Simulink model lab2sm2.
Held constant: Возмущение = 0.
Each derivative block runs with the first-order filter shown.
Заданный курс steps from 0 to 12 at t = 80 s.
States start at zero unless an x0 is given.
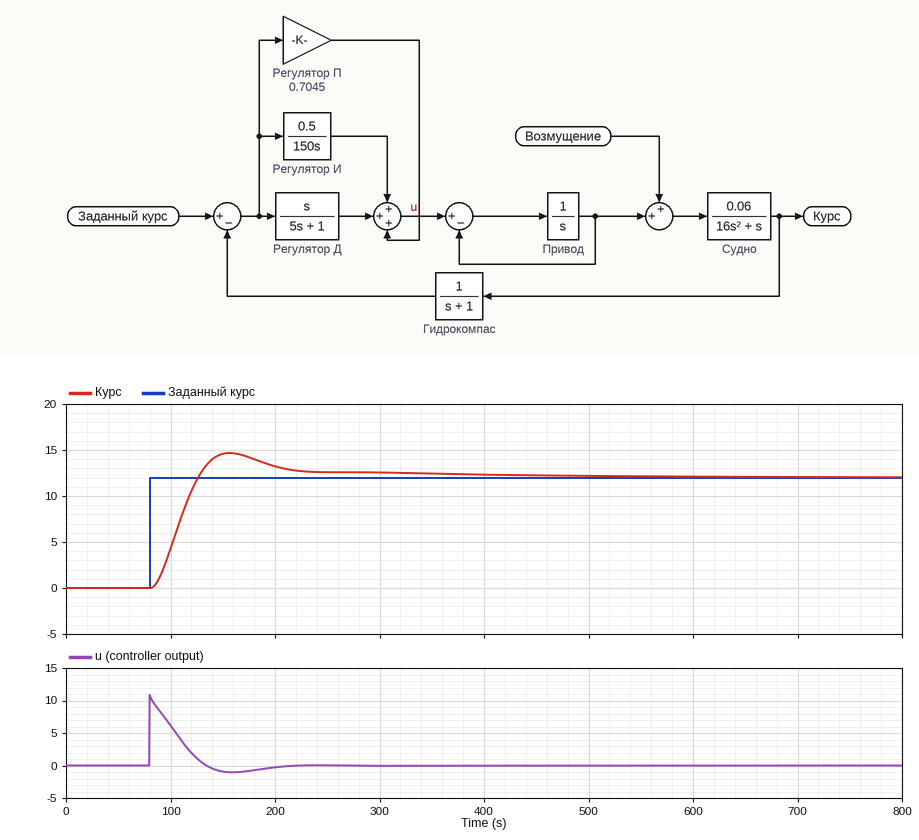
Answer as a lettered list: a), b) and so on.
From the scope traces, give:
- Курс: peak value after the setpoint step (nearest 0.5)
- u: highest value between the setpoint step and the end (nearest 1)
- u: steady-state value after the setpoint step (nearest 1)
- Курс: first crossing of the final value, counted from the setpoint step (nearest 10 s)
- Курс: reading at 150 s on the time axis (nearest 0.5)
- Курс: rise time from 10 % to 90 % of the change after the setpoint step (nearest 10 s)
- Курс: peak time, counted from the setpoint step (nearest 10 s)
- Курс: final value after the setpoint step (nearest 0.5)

a) 14.5
b) 11
c) 0
d) 50 s
e) 14.5
f) 30 s
g) 80 s
h) 12.0
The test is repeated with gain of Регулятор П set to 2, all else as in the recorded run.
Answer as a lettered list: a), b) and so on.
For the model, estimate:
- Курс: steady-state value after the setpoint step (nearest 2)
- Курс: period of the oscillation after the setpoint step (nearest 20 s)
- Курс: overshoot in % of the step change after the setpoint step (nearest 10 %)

a) 12
b) 80 s
c) 40 %
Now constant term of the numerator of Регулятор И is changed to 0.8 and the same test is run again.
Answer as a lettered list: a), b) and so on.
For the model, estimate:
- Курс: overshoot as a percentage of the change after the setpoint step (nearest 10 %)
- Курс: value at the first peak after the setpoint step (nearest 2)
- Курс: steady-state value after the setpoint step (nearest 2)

a) 30 %
b) 16
c) 12
